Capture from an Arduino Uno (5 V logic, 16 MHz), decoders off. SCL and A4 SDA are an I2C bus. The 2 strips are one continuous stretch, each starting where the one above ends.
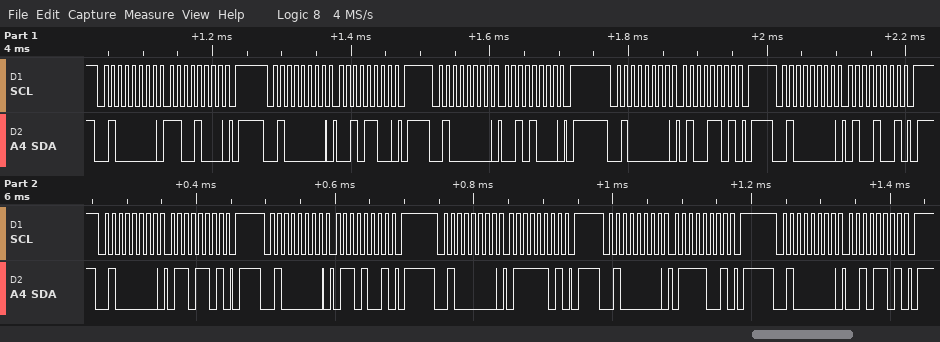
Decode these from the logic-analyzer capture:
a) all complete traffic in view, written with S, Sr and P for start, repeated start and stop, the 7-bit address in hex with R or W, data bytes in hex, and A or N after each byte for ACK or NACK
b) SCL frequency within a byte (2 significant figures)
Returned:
S 20W A C8 A P S 20W A 2C A P S 20W A 28 A P S 20W A 4D A P S 20W A 49 A P S 20W A 6D A P S 20W A 69 A P S 20W A 7D A P S 20W A 79 A P S 20W A 2D A P
100 kHz
